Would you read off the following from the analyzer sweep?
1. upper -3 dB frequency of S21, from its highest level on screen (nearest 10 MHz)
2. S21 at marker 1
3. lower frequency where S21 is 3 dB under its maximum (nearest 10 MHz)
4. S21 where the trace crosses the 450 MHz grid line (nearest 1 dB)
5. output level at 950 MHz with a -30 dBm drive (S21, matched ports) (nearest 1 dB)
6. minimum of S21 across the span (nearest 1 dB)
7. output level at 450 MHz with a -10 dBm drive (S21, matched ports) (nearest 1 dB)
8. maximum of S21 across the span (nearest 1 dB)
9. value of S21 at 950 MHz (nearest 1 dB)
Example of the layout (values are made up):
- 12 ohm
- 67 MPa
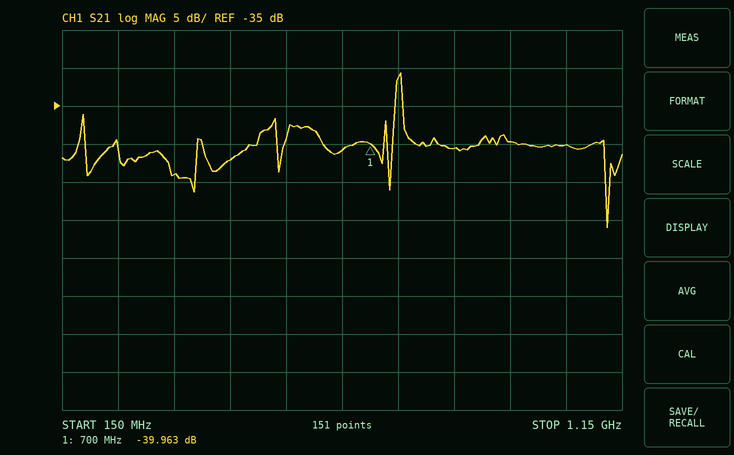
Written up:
- 760 MHz
- -39.963 dB
- 750 MHz
- -42 dB
- -70 dBm
- -51 dB
- -52 dBm
- -31 dB
- -40 dB
